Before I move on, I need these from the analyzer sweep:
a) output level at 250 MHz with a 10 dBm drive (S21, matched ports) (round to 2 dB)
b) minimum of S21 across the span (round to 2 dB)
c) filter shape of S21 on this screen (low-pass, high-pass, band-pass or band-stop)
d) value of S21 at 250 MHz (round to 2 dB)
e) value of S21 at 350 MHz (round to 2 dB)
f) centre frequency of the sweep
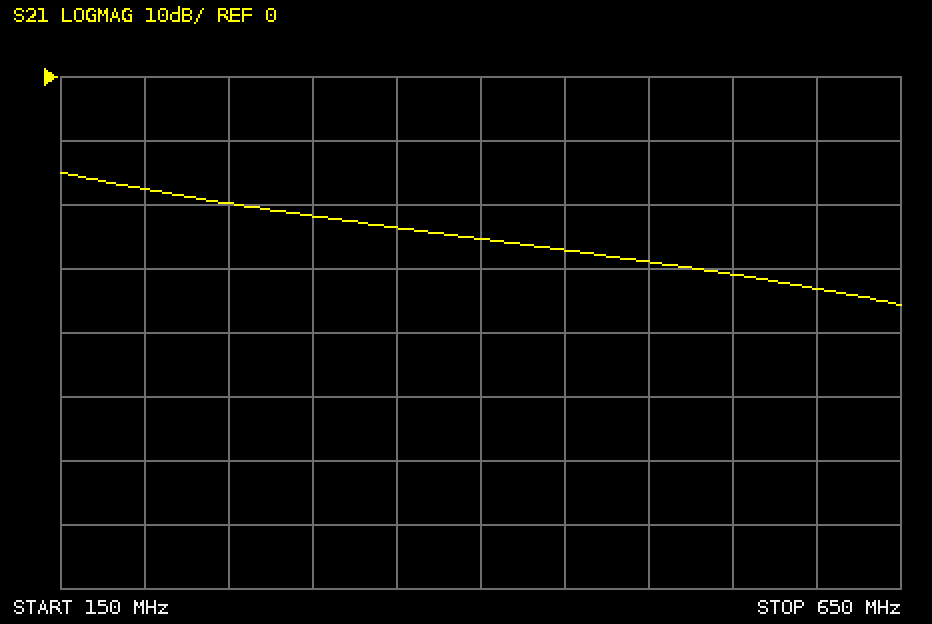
-10 dBm
-36 dB
low-pass
-20 dB
-24 dB
400 MHz
